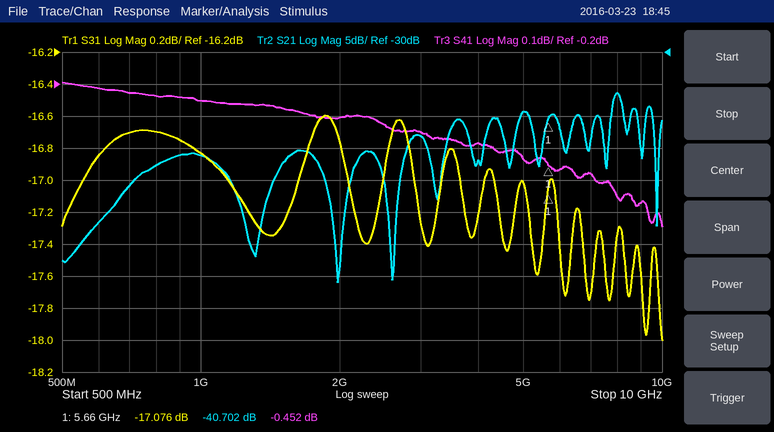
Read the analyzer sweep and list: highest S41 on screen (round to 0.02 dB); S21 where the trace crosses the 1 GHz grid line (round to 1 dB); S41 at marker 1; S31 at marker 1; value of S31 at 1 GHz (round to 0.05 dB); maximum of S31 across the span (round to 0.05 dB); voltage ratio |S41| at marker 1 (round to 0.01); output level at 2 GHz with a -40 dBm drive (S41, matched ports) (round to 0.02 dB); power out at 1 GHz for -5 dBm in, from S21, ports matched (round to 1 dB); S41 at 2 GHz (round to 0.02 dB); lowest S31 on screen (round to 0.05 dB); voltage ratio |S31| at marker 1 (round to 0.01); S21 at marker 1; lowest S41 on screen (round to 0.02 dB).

-0.20 dB
-46 dB
-0.452 dB
-17.076 dB
-16.85 dB
-16.60 dB
0.95
-40.30 dBm
-51 dBm
-0.30 dB
-18.00 dB
0.14
-40.702 dB
-0.64 dB
